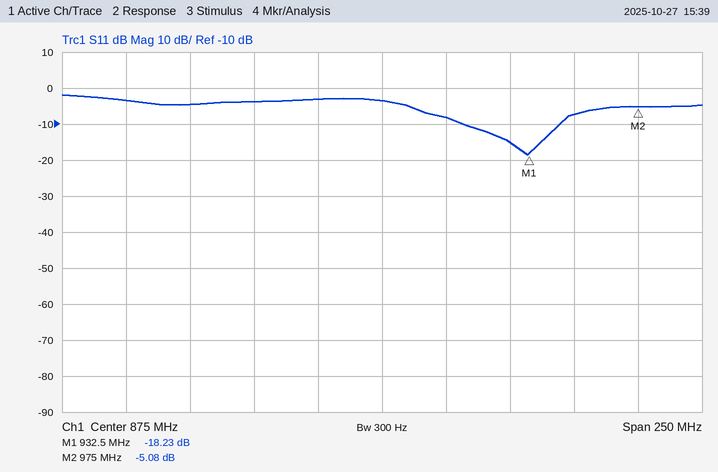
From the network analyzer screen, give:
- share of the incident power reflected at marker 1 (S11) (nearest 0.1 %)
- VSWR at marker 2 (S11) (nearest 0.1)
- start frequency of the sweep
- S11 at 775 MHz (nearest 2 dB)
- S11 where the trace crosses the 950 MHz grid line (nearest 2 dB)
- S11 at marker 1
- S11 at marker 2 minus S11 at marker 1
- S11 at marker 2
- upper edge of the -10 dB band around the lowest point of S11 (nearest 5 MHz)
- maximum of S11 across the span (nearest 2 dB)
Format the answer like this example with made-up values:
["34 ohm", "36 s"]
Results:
["1.5 %", "3.5", "750 MHz", "-4 dB", "-8 dB", "-18.23 dB", "13.15 dB", "-5.08 dB", "945 MHz", "-2 dB"]
